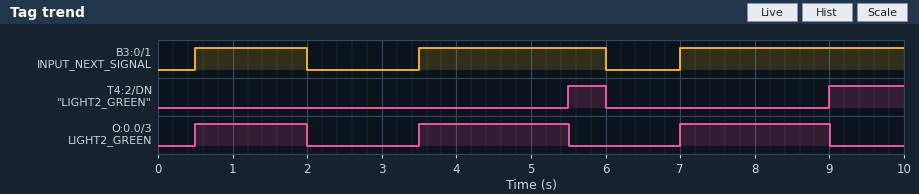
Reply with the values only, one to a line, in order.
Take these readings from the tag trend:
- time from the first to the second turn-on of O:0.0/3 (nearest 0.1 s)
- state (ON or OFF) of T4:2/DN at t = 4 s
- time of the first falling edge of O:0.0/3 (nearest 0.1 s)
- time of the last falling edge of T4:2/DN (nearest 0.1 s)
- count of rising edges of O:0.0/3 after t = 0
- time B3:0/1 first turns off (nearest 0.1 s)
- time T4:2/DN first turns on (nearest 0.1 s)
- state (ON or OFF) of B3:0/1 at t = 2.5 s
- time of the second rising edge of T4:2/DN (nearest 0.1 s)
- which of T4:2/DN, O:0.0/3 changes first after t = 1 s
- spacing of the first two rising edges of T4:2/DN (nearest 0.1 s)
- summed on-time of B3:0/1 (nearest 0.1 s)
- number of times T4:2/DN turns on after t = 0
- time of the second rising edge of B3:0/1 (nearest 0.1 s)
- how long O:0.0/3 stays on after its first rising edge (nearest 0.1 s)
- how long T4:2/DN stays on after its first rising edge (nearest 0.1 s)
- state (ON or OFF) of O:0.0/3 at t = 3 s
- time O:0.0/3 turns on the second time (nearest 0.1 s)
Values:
3.0 s
OFF
2.0 s
6.0 s
3
2.0 s
5.5 s
OFF
9.0 s
O:0.0/3
3.5 s
7.0 s
2
3.5 s
1.5 s
0.5 s
OFF
3.5 s
